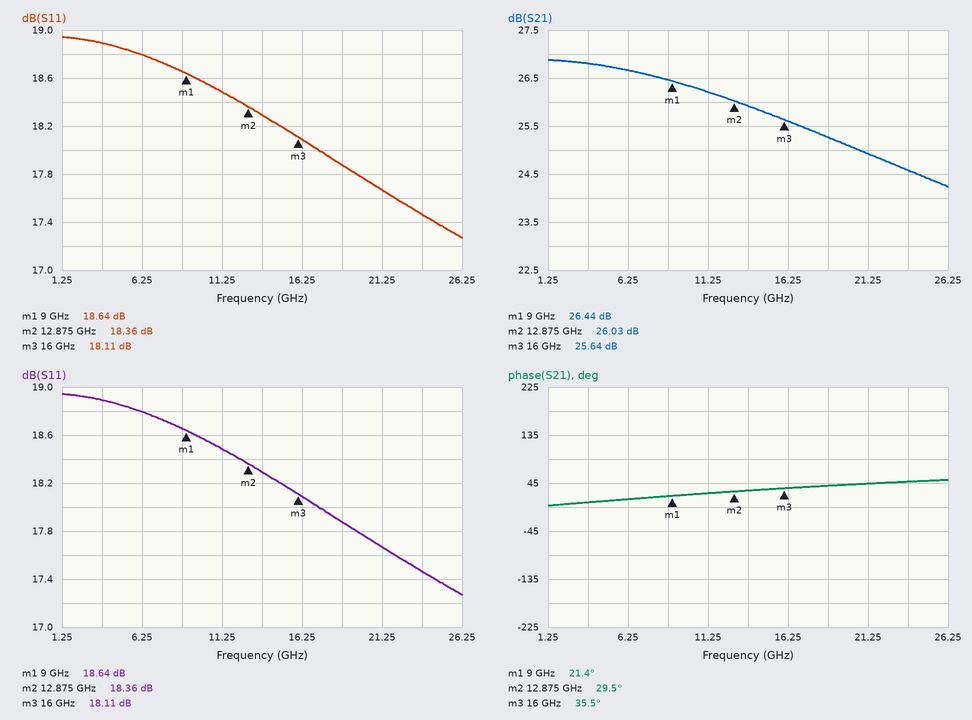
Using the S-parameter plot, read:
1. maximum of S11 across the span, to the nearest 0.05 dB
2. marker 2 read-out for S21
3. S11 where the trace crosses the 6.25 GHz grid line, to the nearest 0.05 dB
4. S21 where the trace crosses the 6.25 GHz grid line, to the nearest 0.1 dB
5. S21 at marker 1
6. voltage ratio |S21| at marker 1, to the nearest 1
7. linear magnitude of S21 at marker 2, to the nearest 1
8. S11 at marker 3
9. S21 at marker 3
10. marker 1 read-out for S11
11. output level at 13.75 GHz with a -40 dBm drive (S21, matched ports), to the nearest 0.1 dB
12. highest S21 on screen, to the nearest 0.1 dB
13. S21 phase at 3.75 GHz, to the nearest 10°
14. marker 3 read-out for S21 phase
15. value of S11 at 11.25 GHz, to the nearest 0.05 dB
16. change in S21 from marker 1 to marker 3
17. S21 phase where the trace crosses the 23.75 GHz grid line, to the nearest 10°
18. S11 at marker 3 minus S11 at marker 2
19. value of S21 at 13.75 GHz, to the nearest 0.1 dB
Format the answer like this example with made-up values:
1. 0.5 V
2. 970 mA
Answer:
1. 18.95 dB
2. 26.03 dB
3. 18.80 dB
4. 26.7 dB
5. 26.44 dB
6. 21
7. 20
8. 18.11 dB
9. 25.64 dB
10. 18.64 dB
11. -14.1 dBm
12. 26.9 dB
13. 10°
14. 35.5°
15. 18.50 dB
16. -0.80 dB
17. 50°
18. -0.25 dB
19. 25.9 dB
